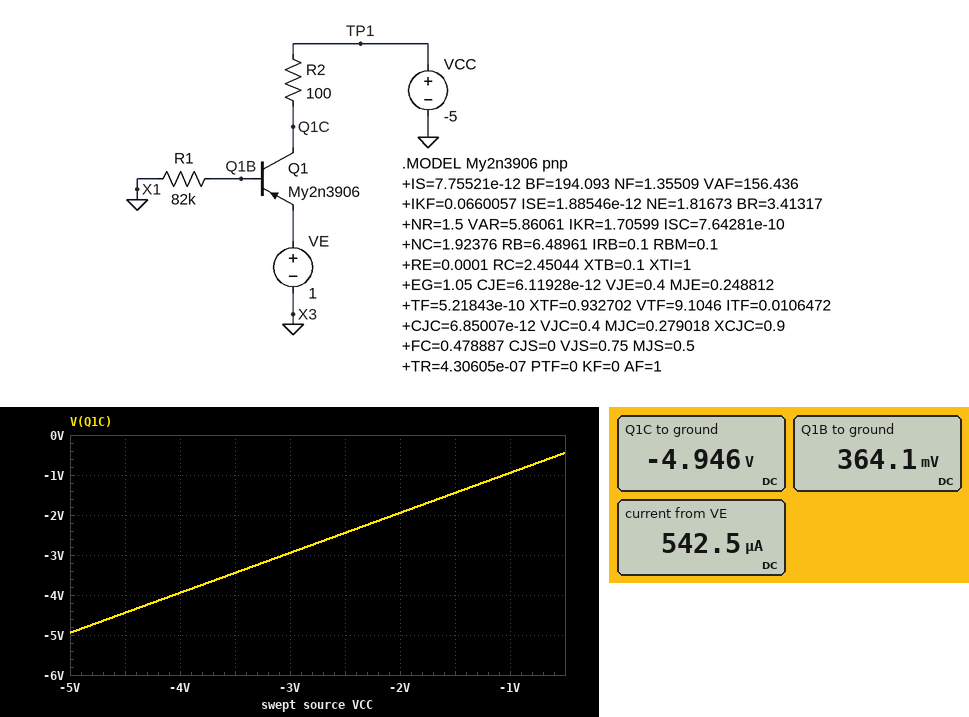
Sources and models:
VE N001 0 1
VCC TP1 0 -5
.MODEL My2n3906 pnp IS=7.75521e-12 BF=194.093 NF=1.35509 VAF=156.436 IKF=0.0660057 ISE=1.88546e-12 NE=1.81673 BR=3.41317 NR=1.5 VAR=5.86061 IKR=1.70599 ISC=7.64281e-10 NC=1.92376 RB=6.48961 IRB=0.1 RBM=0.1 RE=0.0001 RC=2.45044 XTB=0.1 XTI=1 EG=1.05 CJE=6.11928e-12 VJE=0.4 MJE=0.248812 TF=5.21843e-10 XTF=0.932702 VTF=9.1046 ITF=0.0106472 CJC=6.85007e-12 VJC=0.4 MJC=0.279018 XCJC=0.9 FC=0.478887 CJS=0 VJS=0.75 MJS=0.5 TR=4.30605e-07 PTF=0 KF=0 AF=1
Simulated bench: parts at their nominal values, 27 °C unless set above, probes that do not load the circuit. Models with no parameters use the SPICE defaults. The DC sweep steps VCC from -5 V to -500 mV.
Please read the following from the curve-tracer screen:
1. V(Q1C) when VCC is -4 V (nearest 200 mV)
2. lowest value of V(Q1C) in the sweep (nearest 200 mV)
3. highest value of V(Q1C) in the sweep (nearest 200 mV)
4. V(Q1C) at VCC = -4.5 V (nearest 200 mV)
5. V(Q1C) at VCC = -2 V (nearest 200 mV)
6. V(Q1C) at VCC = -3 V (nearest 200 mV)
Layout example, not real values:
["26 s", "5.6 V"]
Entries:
["-4.0 V", "-5.0 V", "-400 mV", "-4.4 V", "-2.0 V", "-3.0 V"]
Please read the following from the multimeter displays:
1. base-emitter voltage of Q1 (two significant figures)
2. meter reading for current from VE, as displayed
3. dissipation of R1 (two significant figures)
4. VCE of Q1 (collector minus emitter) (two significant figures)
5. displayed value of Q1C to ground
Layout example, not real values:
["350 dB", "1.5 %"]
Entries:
["-640 mV", "542.5 µA", "1.6 µW", "-5.9 V", "-4.946 V"]
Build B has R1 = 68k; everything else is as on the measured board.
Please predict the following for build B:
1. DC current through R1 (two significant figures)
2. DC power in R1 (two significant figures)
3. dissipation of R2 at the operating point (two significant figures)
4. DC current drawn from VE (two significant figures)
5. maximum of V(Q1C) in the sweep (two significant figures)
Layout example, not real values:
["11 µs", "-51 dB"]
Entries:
["5.3 µA", "1.9 µW", "42 µW", "650 µA", "-440 mV"]
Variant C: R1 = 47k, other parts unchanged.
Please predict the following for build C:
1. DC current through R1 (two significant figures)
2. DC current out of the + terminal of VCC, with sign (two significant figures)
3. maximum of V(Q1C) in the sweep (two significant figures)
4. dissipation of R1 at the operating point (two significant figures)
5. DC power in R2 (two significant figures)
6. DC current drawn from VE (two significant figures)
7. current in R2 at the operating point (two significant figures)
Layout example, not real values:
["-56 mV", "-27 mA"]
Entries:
["7.3 µA", "-920 µA", "-410 mV", "2.5 µW", "84 µW", "930 µA", "920 µA"]
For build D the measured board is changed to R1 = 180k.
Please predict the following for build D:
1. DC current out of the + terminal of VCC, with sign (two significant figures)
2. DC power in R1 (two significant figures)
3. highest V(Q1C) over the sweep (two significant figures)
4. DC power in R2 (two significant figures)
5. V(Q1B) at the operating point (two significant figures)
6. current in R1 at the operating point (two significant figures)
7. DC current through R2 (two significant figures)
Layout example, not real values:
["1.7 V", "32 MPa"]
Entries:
["-250 µA", "850 nW", "-480 mV", "6.2 µW", "390 mV", "2.2 µA", "250 µA"]
